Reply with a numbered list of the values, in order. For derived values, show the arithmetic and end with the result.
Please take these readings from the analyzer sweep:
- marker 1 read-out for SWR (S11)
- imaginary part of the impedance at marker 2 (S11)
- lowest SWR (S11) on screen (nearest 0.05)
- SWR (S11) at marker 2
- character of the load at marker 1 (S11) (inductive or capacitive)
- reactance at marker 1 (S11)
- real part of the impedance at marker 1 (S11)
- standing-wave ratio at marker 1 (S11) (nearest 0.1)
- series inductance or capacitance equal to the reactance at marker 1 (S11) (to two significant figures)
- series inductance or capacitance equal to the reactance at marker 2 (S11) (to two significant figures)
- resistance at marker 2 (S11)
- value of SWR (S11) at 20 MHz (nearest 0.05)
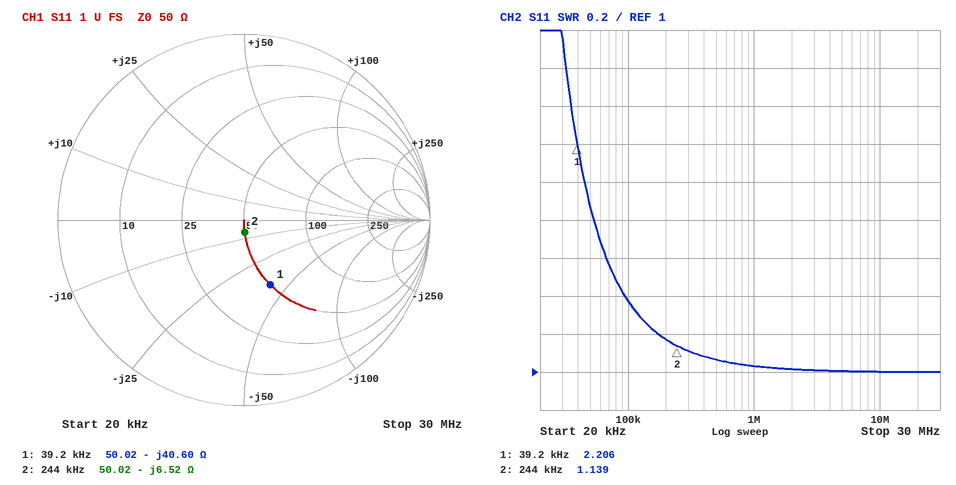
1. 2.206
2. -6.52 Ω
3. 1.00
4. 1.139
5. capacitive
6. -40.60 Ω
7. 50.02 Ω
8. 2.2
9. C = 1/(2π × 39.2 kHz × 40.6 Ω) ≈ 100 nF
10. C = 1/(2π × 244 kHz × 6.52 Ω) ≈ 100 nF
11. 50.02 Ω
12. 1.00
